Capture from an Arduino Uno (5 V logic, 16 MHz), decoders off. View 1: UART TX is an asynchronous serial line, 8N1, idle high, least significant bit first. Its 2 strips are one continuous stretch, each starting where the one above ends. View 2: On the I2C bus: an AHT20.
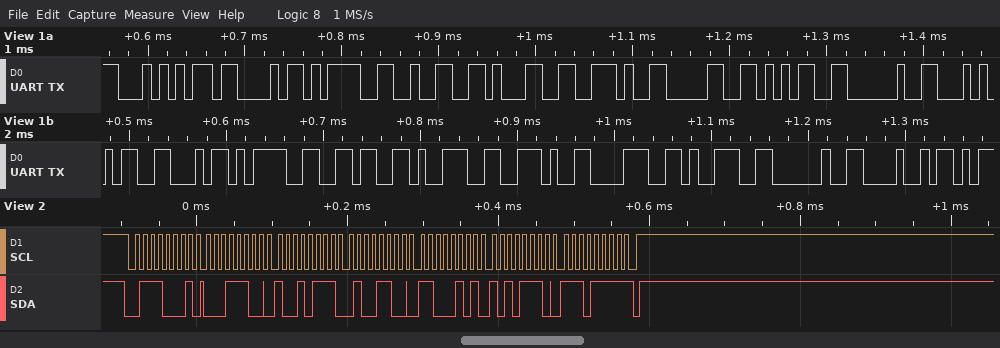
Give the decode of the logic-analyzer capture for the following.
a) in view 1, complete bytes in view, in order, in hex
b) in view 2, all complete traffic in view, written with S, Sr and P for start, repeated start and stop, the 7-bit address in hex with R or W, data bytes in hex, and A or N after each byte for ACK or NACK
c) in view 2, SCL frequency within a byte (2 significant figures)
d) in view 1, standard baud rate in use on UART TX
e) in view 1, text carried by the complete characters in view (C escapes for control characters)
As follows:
54 43 3D 32 31 2E 30 35 20 54 46 3D 36 39 2E 38 39 20 48
S 38R A 1C A 97 A 4C A C5 A AE A EF N P
100 kHz
115200 baud
"TC=21.05 TF=69.89 H"
